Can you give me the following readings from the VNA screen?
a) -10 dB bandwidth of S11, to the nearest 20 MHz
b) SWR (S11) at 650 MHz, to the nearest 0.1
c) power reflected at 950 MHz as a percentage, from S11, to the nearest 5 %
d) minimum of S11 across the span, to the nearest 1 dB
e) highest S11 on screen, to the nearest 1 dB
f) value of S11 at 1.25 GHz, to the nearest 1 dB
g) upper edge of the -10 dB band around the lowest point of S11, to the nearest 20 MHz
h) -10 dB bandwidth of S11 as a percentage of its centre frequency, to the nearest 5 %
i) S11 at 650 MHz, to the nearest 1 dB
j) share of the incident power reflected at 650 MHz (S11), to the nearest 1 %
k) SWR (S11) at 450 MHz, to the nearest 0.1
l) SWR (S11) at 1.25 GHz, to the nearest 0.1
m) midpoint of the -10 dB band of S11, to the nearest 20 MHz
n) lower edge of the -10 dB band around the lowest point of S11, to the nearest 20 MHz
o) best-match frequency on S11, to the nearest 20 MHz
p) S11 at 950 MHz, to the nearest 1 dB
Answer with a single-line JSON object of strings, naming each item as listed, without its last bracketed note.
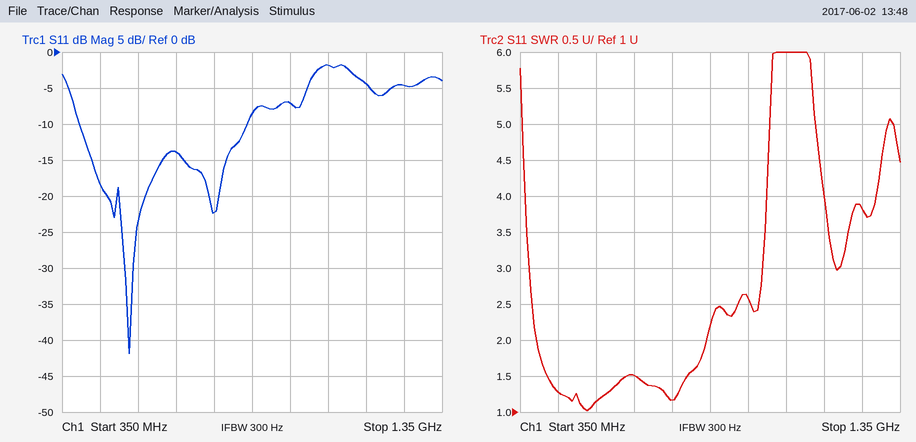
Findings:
{"-10 dB bandwidth of S11, to the nearest 20 MHz": "440 MHz", "SWR (S11) at 650 MHz, to the nearest 0.1": "1.5", "power reflected at 950 MHz as a percentage, from S11, to the nearest 5 %": "20 %", "minimum of S11 across the span, to the nearest 1 dB": "-42 dB", "highest S11 on screen, to the nearest 1 dB": "-2 dB", "value of S11 at 1.25 GHz, to the nearest 1 dB": "-5 dB", "upper edge of the -10 dB band around the lowest point of S11, to the nearest 20 MHz": "840 MHz", "-10 dB bandwidth of S11 as a percentage of its centre frequency, to the nearest 5 %": "70 %", "S11 at 650 MHz, to the nearest 1 dB": "-14 dB", "share of the incident power reflected at 650 MHz (S11), to the nearest 1 %": "4 %", "SWR (S11) at 450 MHz, to the nearest 0.1": "1.3", "SWR (S11) at 1.25 GHz, to the nearest 0.1": "3.8", "midpoint of the -10 dB band of S11, to the nearest 20 MHz": "620 MHz", "lower edge of the -10 dB band around the lowest point of S11, to the nearest 20 MHz": "400 MHz", "best-match frequency on S11, to the nearest 20 MHz": "520 MHz", "S11 at 950 MHz, to the nearest 1 dB": "-7 dB"}
